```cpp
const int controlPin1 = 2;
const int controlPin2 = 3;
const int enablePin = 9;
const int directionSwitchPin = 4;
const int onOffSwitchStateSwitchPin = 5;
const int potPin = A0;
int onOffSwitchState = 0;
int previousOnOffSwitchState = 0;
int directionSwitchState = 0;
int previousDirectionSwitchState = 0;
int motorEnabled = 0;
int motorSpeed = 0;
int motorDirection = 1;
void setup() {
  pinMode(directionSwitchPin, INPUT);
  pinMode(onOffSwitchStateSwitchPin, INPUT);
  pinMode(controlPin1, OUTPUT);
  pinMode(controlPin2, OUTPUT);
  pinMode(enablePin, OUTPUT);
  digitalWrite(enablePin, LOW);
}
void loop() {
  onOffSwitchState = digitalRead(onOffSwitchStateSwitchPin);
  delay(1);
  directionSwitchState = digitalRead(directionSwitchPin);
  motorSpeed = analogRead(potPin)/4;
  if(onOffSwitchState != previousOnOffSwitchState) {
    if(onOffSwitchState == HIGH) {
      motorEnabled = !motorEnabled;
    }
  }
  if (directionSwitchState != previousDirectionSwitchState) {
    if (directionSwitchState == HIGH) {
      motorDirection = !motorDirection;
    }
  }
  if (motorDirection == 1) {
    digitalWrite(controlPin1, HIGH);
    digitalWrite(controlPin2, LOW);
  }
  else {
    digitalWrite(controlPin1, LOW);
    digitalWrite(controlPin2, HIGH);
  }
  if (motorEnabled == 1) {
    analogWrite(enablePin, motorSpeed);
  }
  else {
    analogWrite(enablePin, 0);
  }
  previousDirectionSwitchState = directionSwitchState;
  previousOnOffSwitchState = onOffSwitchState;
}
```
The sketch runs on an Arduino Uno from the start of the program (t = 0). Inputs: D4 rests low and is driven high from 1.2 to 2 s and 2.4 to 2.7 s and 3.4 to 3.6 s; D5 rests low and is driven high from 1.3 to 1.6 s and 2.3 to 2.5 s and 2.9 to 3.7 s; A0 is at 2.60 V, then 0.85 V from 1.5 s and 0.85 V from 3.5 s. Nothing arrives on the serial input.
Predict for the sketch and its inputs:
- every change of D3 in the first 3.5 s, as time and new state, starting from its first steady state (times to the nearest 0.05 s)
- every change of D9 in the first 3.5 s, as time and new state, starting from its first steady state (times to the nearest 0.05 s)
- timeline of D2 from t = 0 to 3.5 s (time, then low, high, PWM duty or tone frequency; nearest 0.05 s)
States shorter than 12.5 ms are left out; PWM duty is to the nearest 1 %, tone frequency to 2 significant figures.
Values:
0 s low; 1.2 s high; 2.4 s low; 3.4 s high
0 s low; 1.3 s PWM 52 %; 1.5 s PWM 17 %; 2.3 s low; 2.9 s PWM 17 %
0 s high; 1.2 s low; 2.4 s high; 3.4 s low
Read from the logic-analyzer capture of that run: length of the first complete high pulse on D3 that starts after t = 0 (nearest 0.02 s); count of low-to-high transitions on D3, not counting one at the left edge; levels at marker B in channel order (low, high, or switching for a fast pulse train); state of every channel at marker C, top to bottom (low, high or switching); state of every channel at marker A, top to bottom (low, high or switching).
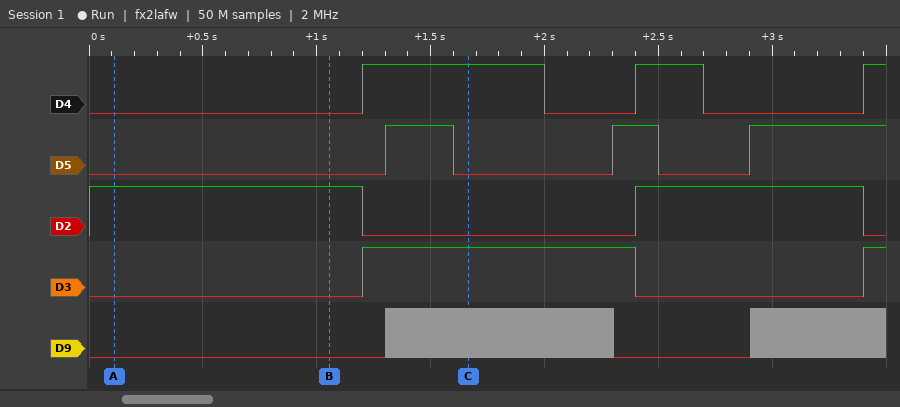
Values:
1.20 s
2
D4 low, D5 low, D2 high, D3 low, D9 low
D4 high, D5 low, D2 low, D3 high, D9 switching
D4 low, D5 low, D2 high, D3 low, D9 low
